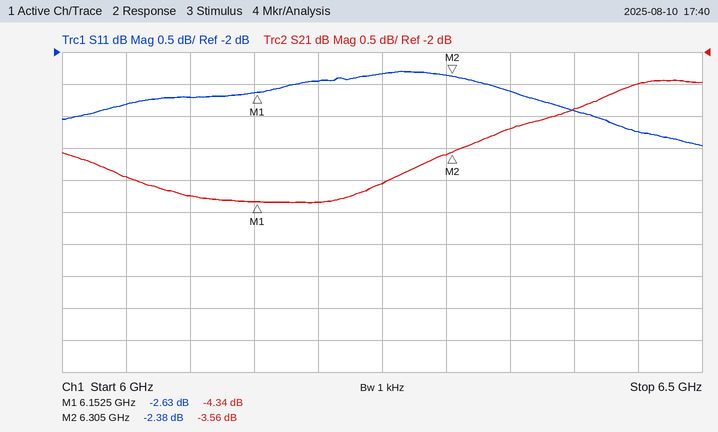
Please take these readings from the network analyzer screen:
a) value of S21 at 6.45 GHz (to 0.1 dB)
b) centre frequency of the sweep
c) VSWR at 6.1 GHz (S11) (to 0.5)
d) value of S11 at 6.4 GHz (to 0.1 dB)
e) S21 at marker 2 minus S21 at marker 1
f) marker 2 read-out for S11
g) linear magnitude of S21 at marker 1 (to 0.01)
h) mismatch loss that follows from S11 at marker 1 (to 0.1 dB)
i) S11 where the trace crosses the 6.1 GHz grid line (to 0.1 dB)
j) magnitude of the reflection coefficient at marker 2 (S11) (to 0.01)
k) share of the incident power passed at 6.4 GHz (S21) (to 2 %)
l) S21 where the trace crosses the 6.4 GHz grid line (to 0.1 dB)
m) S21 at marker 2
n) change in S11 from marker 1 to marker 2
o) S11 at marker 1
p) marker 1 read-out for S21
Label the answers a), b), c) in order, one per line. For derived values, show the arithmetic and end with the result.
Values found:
a) -2.5 dB
b) 6.25 GHz
c) |Γ| = 10^(-2.7/20) = 0.7328; VSWR = (1 + 0.7328)/(1 − 0.7328) ≈ 6.5
d) -2.9 dB
e) -3.56 − (-4.34) = 0.78 dB
f) -2.38 dB
g) 10^(-4.34/20) ≈ 0.61
h) −10 log10(1 − 10^(-2.63/10)) ≈ 3.4 dB
i) -2.7 dB
j) 10^(-2.38/20) ≈ 0.76
k) 10^(-2.9/10) ≈ 51.3 %, so 52 % to the nearest 2 %
l) -2.9 dB
m) -3.56 dB
n) -2.38 − (-2.63) = 0.25 dB
o) -2.63 dB
p) -4.34 dB
